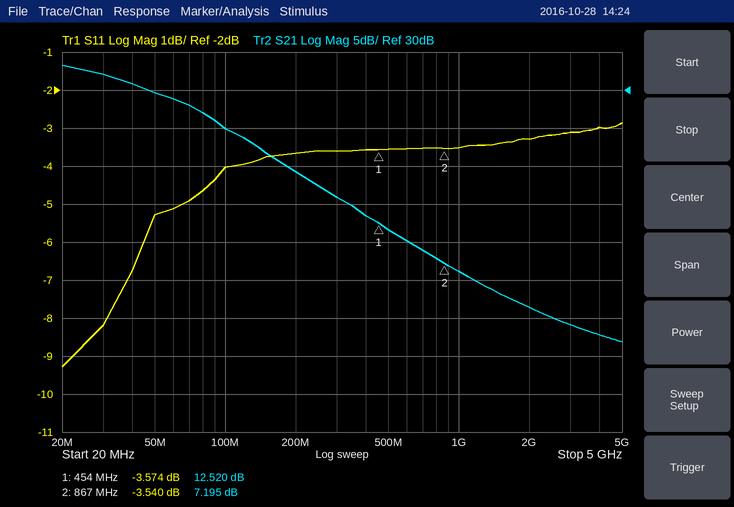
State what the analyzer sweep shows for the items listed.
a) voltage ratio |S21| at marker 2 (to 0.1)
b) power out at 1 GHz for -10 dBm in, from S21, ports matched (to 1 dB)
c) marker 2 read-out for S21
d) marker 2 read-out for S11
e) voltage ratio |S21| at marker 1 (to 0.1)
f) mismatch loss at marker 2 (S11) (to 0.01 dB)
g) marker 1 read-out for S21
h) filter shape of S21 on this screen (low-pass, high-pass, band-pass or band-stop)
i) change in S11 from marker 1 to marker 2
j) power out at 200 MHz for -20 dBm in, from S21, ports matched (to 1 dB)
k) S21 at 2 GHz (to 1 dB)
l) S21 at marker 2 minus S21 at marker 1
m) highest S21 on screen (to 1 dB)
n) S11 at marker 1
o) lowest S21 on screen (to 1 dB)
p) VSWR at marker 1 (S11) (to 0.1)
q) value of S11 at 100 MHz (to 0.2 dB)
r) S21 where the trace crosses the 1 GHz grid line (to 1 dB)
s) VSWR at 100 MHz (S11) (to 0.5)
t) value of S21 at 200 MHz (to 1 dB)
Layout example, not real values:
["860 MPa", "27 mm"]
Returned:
["2.3", "-4 dBm", "7.195 dB", "-3.540 dB", "4.2", "2.54 dB", "12.520 dB", "low-pass", "0.034 dB", "-1 dBm", "1 dB", "-5.325 dB", "33 dB", "-3.574 dB", "-3 dB", "4.9", "-4.0 dB", "6 dB", "4.5", "19 dB"]
